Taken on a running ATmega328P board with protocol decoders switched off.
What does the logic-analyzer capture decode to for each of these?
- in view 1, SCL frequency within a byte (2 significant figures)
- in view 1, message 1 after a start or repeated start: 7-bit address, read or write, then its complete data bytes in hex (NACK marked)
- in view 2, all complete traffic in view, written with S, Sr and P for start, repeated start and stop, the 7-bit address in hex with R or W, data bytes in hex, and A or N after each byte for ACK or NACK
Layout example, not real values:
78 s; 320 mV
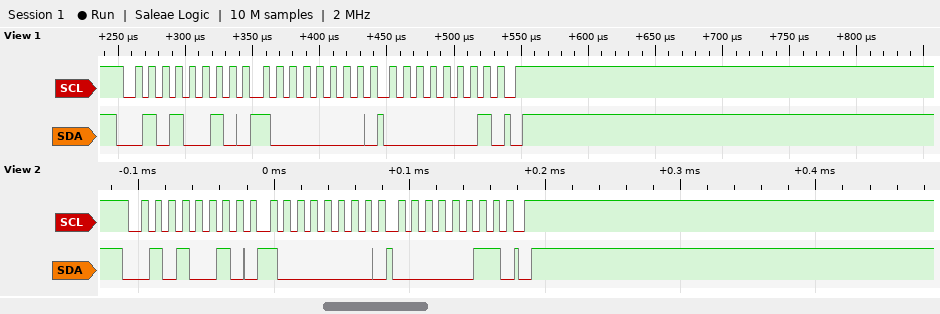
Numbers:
100 kHz; 0x29 write: 80 01; S 29W A 80 A 03 A P
